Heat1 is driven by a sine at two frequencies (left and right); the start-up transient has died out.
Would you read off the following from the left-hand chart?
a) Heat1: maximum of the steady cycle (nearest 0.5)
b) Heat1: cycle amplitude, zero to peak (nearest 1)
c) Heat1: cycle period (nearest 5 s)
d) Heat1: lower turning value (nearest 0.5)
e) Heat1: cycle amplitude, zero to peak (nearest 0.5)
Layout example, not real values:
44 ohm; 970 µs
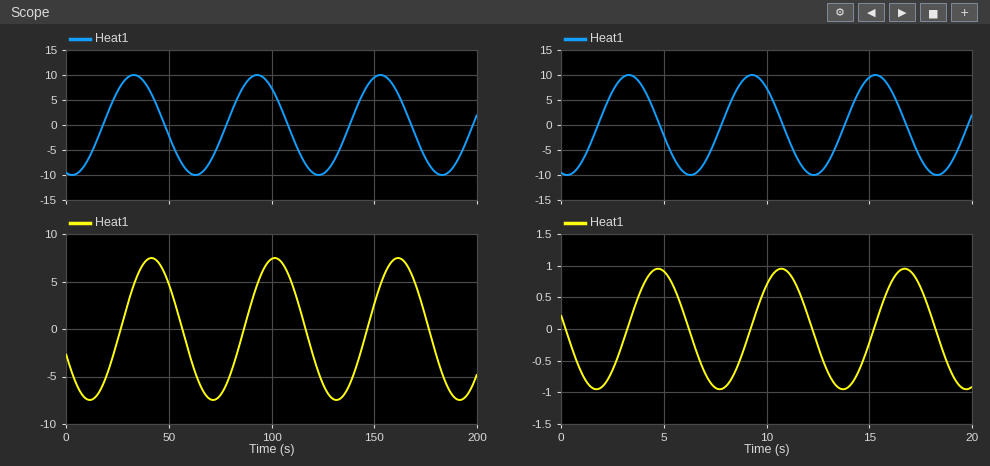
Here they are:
7.5; 10; 60 s; -7.5; 7.5
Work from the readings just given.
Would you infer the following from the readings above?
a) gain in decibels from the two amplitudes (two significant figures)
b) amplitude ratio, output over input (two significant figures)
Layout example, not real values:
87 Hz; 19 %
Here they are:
-2.5 dB; 0.75
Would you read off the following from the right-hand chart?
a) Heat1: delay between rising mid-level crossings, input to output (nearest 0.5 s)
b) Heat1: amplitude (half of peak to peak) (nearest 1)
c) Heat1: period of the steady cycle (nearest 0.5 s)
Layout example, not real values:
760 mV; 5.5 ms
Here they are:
1.5 s; 10; 6.0 s
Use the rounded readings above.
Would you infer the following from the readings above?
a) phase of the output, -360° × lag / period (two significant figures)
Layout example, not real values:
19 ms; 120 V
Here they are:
-90°
